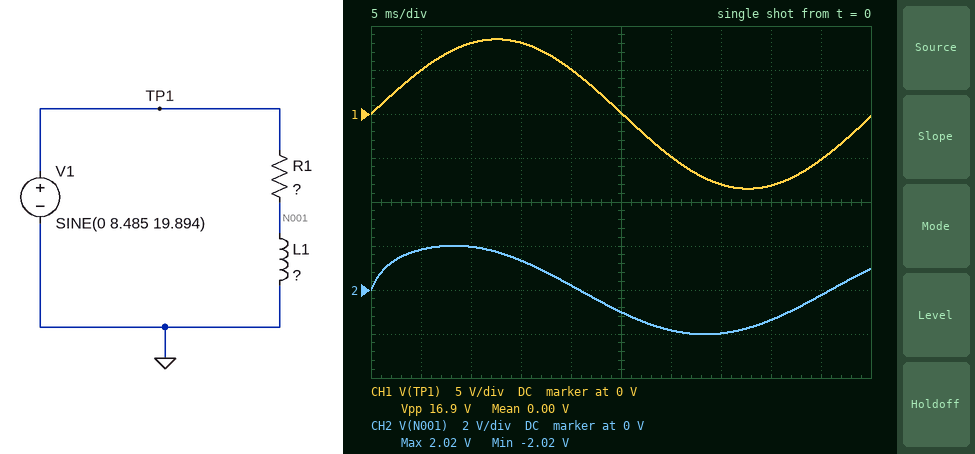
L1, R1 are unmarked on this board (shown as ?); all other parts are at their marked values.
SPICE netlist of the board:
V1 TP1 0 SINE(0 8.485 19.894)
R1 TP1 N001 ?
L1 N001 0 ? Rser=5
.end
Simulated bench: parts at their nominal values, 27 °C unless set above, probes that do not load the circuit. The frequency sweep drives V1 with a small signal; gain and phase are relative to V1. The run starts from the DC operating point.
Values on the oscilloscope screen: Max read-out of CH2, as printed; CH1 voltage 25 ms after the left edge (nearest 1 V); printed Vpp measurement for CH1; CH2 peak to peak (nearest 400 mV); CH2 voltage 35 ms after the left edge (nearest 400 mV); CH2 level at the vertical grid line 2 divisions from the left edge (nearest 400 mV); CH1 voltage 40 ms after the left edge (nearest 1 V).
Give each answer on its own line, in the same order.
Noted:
2.02 V
0 V
16.9 V
4.0 V
-2.0 V
2.0 V
-8 V
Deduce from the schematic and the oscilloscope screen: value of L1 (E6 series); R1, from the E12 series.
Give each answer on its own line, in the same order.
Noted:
33 mH
22 Ω
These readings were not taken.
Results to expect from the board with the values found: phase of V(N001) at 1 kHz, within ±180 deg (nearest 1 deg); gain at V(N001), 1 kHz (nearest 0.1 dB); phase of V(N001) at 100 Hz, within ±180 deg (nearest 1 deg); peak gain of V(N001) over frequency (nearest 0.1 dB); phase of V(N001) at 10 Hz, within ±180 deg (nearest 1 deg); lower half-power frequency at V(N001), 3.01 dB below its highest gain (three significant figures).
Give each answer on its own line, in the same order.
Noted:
6 deg
-0.1 dB
39 deg
0 dB
18 deg
126 Hz
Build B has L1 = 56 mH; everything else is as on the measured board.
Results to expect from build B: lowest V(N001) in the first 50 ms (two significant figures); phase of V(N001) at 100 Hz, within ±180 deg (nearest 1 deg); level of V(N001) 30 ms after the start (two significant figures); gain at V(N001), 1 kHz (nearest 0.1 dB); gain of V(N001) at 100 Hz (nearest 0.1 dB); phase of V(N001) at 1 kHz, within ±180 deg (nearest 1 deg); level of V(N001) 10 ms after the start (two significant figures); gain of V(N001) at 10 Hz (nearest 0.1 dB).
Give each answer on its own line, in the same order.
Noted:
-2.6 V
29 deg
-2.5 V
0 dB
-1.9 dB
4 deg
2.4 V
-13.0 dB
